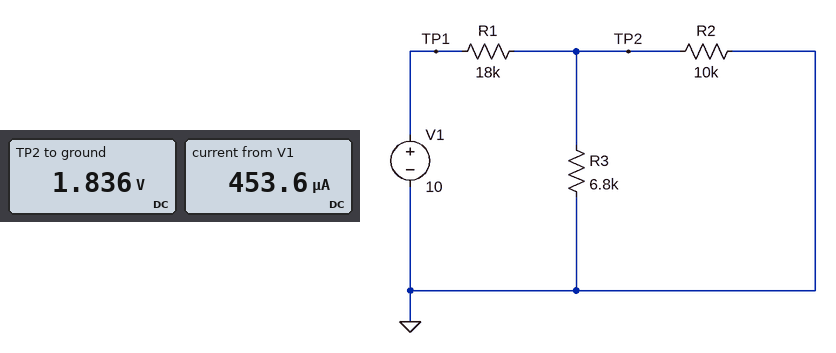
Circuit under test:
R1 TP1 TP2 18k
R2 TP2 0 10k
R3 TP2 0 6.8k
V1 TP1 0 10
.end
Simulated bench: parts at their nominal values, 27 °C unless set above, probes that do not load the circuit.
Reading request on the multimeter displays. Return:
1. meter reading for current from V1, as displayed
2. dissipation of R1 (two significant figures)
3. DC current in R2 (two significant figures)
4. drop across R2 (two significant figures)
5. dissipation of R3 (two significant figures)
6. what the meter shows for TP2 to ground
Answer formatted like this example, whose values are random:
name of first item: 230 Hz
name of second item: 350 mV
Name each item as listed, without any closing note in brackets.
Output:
meter reading for current from V1, as displayed: 453.6 µA
dissipation of R1: 3.7 mW
DC current in R2: 180 µA
drop across R2: 1.8 V
dissipation of R3: 500 µW
what the meter shows for TP2 to ground: 1.836 V
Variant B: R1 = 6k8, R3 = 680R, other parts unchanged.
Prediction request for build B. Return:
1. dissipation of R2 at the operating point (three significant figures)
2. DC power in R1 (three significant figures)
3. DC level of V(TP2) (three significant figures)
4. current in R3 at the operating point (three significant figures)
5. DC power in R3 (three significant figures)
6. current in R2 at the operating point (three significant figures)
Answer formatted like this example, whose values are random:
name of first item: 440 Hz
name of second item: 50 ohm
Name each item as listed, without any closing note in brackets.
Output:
dissipation of R2 at the operating point: 73.3 µW
DC power in R1: 12.3 mW
DC level of V(TP2): 856 mV
current in R3 at the operating point: 1.26 mA
DC power in R3: 1.08 mW
current in R2 at the operating point: 85.6 µA
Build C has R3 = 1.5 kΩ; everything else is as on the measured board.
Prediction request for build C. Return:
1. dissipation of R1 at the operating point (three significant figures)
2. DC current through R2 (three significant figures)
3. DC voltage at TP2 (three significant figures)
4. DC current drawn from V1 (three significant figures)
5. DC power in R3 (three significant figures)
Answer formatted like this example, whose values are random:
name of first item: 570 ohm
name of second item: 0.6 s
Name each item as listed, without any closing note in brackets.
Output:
dissipation of R1 at the operating point: 4.83 mW
DC current through R2: 67.6 µA
DC voltage at TP2: 676 mV
DC current drawn from V1: 518 µA
DC power in R3: 304 µW
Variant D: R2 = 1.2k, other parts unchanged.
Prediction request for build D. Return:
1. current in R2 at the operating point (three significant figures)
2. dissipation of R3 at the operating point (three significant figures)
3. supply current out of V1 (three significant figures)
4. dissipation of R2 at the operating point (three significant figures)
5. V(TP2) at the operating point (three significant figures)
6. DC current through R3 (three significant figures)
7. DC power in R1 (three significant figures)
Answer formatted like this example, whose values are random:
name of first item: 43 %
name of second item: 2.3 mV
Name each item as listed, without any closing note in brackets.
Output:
current in R2 at the operating point: 447 µA
dissipation of R3 at the operating point: 42.3 µW
supply current out of V1: 526 µA
dissipation of R2 at the operating point: 240 µW
V(TP2) at the operating point: 536 mV
DC current through R3: 78.9 µA
DC power in R1: 4.98 mW
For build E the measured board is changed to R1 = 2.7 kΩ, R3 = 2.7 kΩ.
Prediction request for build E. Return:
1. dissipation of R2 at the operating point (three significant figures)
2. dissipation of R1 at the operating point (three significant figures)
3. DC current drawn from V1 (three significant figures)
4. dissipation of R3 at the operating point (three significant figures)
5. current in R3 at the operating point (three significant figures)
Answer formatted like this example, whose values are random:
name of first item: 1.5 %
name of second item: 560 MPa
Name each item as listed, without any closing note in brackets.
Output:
dissipation of R2 at the operating point: 1.94 mW
dissipation of R1 at the operating point: 11.6 mW
DC current drawn from V1: 2.07 mA
dissipation of R3 at the operating point: 7.19 mW
current in R3 at the operating point: 1.63 mA
